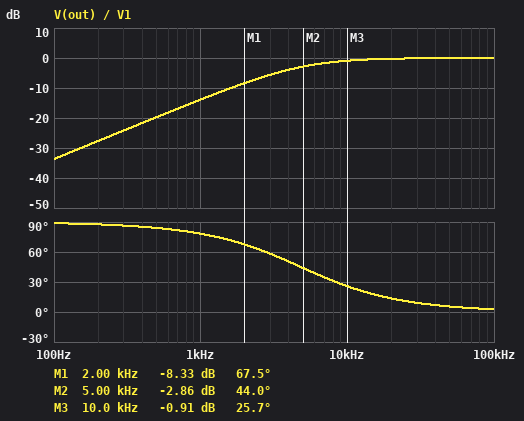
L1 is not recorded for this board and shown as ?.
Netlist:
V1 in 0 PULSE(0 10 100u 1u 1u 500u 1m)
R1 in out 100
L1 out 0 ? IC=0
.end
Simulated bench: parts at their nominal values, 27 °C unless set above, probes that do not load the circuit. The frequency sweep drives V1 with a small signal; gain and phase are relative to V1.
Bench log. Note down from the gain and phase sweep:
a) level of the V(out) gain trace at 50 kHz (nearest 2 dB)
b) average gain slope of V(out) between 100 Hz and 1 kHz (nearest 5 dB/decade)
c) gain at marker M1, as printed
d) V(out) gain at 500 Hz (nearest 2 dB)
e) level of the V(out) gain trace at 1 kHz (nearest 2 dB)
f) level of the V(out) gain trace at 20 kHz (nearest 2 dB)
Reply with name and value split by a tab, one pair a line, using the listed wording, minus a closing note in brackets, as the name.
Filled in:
level of the V(out) gain trace at 50 kHz	0 dB
average gain slope of V(out) between 100 Hz and 1 kHz	20 dB/decade
gain at marker M1, as printed	-8.33 dB
V(out) gain at 500 Hz	-20 dB
level of the V(out) gain trace at 1 kHz	-14 dB
level of the V(out) gain trace at 20 kHz	0 dB
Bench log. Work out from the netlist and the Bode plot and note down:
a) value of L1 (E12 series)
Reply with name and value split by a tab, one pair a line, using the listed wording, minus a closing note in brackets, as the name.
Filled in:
value of L1	3.3 mH
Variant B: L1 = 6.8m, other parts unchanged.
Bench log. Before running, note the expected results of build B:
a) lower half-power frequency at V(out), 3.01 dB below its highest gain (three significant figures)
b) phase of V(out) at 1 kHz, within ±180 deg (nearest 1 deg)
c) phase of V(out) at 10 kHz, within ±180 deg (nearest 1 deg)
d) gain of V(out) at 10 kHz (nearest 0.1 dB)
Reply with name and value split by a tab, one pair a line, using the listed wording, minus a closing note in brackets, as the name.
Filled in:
lower half-power frequency at V(out), 3.01 dB below its highest gain	2.34 kHz
phase of V(out) at 1 kHz, within ±180 deg	67 deg
phase of V(out) at 10 kHz, within ±180 deg	13 deg
gain of V(out) at 10 kHz	-0.2 dB
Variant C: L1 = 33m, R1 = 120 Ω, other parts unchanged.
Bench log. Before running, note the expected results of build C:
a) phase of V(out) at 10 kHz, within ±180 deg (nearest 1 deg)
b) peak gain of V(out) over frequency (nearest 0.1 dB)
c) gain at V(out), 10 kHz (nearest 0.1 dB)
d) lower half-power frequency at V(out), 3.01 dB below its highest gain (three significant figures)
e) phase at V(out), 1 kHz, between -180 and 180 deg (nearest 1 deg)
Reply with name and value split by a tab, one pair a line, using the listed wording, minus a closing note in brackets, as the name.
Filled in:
phase of V(out) at 10 kHz, within ±180 deg	3 deg
peak gain of V(out) over frequency	0 dB
gain at V(out), 10 kHz	0 dB
lower half-power frequency at V(out), 3.01 dB below its highest gain	579 Hz
phase at V(out), 1 kHz, between -180 and 180 deg	30 deg
